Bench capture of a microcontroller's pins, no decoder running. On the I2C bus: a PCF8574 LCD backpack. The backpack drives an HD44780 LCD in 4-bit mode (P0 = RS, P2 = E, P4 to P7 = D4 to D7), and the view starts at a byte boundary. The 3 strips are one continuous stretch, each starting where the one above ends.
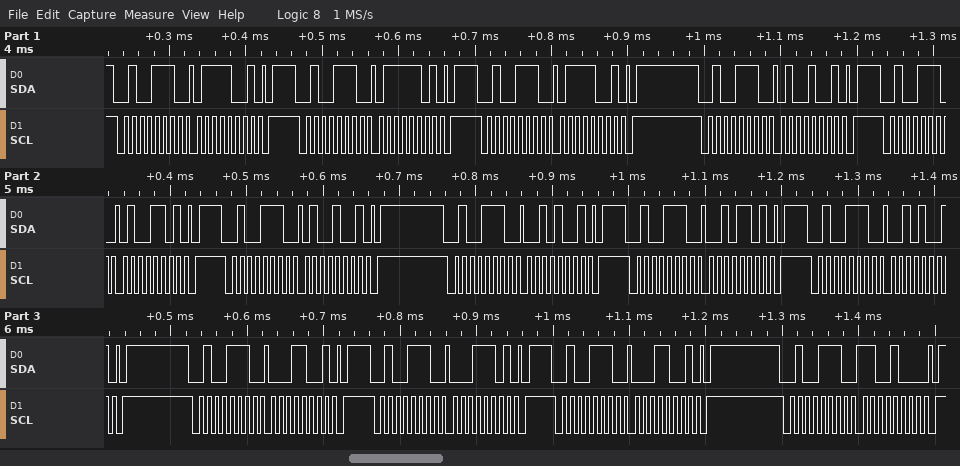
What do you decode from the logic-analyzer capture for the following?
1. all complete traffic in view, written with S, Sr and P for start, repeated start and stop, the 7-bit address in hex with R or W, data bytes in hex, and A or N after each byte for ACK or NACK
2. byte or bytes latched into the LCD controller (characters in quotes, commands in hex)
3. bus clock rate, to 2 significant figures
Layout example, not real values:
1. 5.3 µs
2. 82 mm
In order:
1. S 27W A 79 A P S 27W A 7D A P S 27W A 79 A P S 27W A 49 A P S 27W A 4D A P S 27W A 49 A P S 27W A 29 A P S 27W A 2D A P S 27W A 29 A P S 27W A 19 A P S 27W A 1D A P S 27W A 19 A P S 27W A C8 A P
2. 't' '!'
3. 100 kHz
